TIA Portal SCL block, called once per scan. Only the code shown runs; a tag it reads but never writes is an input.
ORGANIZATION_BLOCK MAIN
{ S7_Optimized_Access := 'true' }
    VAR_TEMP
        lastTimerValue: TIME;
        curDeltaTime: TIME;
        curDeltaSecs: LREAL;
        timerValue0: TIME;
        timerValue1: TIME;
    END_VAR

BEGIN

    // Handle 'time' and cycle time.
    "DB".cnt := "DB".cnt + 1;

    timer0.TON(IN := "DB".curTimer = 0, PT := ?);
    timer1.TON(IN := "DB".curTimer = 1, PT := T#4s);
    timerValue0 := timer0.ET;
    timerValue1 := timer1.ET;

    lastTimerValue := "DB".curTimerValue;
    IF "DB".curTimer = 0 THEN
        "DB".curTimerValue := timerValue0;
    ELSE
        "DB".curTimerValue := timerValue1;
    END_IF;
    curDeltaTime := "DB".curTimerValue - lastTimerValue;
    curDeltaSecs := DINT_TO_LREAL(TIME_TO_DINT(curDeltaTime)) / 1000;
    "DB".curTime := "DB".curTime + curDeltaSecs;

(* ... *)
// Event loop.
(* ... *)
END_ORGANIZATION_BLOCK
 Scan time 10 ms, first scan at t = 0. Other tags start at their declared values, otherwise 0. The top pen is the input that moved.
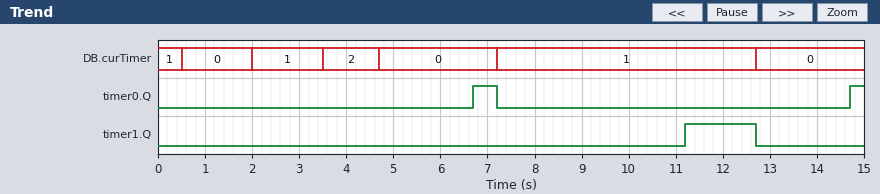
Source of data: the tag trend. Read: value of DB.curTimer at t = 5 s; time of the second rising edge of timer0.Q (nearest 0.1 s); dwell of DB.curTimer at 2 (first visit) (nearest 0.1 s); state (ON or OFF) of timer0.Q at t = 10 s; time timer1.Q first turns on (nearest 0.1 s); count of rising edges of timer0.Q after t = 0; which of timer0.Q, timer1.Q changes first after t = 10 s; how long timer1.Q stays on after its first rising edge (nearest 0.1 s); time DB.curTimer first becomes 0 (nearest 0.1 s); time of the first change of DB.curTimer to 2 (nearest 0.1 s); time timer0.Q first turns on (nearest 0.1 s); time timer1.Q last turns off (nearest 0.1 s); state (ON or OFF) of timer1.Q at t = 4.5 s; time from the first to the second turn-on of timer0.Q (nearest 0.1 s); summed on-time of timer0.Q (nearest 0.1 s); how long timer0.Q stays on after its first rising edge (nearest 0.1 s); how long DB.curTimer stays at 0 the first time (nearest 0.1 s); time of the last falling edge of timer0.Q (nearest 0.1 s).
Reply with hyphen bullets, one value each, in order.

- 0
- 14.7 s
- 1.2 s
- OFF
- 11.2 s
- 2
- timer1.Q
- 1.5 s
- 0.5 s
- 3.5 s
- 6.7 s
- 12.7 s
- OFF
- 8.0 s
- 0.8 s
- 0.5 s
- 1.5 s
- 7.2 s
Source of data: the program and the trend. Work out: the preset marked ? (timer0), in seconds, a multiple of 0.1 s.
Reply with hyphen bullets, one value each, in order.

- 2.0 s
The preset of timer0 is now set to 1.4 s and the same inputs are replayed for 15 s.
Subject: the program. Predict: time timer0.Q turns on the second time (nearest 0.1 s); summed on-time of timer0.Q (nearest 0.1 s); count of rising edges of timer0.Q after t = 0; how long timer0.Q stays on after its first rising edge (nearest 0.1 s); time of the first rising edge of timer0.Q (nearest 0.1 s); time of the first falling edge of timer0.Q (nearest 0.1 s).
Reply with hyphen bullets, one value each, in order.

- 6.1 s
- 2.1 s
- 3
- 0.1 s
- 1.9 s
- 2.0 s
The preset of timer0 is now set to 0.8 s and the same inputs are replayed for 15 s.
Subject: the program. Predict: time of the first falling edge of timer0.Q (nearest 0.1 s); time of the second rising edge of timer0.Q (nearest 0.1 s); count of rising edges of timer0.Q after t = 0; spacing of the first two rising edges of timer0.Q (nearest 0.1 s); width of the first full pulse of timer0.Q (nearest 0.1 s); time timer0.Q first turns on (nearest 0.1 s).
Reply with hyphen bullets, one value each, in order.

- 2.0 s
- 5.5 s
- 3
- 4.2 s
- 0.7 s
- 1.3 s
